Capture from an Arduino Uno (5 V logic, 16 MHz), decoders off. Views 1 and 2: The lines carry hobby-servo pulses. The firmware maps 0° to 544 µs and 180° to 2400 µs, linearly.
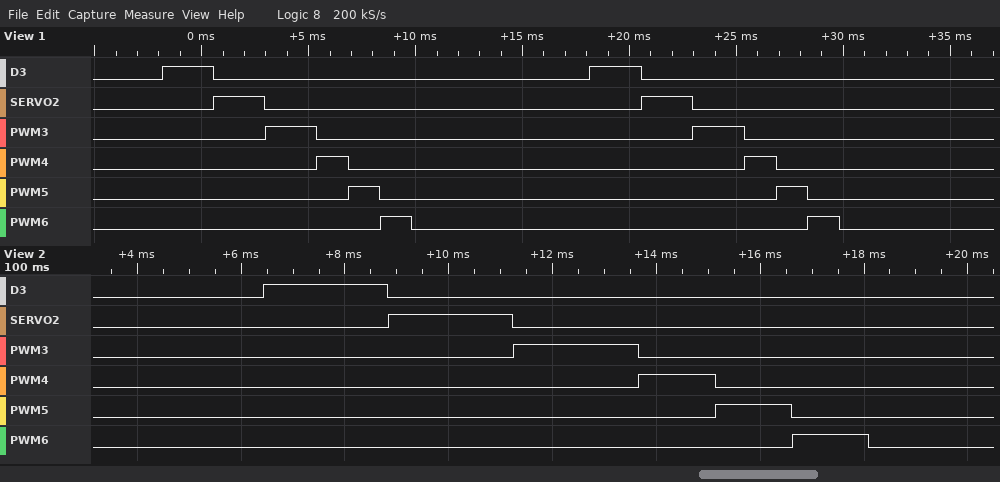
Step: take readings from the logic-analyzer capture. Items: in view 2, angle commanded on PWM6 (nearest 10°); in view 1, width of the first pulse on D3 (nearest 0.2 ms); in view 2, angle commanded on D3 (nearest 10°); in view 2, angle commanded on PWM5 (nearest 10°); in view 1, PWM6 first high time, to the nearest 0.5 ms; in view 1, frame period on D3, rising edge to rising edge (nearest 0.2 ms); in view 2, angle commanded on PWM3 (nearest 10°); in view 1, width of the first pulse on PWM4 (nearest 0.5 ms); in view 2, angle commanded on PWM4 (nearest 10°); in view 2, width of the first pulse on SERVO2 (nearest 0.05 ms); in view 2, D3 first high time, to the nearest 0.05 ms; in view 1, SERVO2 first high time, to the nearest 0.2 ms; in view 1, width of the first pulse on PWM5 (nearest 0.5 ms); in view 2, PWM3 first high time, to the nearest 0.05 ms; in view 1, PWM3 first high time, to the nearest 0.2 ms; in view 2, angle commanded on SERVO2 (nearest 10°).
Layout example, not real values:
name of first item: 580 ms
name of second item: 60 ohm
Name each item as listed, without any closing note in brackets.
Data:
in view 2, angle commanded on PWM6: 90°
in view 1, width of the first pulse on D3: 2.4 ms
in view 2, angle commanded on D3: 180°
in view 2, angle commanded on PWM5: 90°
in view 1, PWM6 first high time, to the nearest 0.5 ms: 1.5 ms
in view 1, frame period on D3, rising edge to rising edge: 20.0 ms
in view 2, angle commanded on PWM3: 180°
in view 1, width of the first pulse on PWM4: 1.5 ms
in view 2, angle commanded on PWM4: 90°
in view 2, width of the first pulse on SERVO2: 2.40 ms
in view 2, D3 first high time, to the nearest 0.05 ms: 2.40 ms
in view 1, SERVO2 first high time, to the nearest 0.2 ms: 2.4 ms
in view 1, width of the first pulse on PWM5: 1.5 ms
in view 2, PWM3 first high time, to the nearest 0.05 ms: 2.40 ms
in view 1, PWM3 first high time, to the nearest 0.2 ms: 2.4 ms
in view 2, angle commanded on SERVO2: 180°
